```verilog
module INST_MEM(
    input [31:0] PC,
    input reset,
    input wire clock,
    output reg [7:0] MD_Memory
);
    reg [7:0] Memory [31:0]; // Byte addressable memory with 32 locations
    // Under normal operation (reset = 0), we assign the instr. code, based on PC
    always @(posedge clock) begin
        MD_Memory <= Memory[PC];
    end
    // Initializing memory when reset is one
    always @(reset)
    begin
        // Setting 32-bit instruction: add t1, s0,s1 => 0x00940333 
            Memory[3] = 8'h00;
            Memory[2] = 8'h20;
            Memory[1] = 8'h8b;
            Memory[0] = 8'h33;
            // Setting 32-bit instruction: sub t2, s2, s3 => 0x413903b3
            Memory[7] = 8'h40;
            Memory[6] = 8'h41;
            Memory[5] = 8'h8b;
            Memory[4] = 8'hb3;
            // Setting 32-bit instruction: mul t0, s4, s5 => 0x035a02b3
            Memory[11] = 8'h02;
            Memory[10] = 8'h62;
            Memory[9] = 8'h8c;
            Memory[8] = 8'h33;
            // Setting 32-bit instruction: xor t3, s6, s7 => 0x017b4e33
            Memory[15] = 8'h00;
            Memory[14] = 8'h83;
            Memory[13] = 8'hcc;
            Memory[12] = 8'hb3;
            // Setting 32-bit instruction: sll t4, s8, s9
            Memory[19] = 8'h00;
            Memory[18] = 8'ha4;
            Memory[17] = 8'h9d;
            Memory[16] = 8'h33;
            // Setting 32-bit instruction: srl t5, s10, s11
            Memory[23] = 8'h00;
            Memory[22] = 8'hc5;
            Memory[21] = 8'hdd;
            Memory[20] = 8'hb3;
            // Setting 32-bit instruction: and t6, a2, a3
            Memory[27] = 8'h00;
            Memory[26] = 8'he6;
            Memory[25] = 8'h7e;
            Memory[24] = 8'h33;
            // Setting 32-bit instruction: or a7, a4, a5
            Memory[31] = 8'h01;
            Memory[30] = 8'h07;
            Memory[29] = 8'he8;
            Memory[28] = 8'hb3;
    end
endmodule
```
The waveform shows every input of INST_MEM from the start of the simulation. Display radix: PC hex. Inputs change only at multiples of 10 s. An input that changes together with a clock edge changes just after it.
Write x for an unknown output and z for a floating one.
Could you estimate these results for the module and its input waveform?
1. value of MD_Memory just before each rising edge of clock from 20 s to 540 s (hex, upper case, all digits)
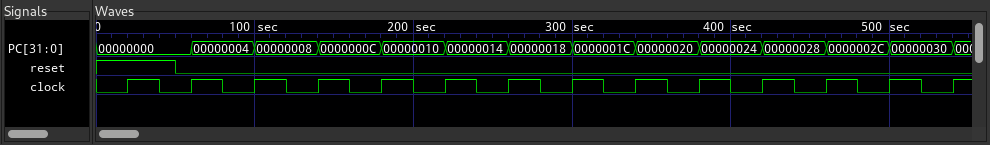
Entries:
x, 33, 33, B3, 33, B3, 33, B3, 33, B3, x, x, x, x
